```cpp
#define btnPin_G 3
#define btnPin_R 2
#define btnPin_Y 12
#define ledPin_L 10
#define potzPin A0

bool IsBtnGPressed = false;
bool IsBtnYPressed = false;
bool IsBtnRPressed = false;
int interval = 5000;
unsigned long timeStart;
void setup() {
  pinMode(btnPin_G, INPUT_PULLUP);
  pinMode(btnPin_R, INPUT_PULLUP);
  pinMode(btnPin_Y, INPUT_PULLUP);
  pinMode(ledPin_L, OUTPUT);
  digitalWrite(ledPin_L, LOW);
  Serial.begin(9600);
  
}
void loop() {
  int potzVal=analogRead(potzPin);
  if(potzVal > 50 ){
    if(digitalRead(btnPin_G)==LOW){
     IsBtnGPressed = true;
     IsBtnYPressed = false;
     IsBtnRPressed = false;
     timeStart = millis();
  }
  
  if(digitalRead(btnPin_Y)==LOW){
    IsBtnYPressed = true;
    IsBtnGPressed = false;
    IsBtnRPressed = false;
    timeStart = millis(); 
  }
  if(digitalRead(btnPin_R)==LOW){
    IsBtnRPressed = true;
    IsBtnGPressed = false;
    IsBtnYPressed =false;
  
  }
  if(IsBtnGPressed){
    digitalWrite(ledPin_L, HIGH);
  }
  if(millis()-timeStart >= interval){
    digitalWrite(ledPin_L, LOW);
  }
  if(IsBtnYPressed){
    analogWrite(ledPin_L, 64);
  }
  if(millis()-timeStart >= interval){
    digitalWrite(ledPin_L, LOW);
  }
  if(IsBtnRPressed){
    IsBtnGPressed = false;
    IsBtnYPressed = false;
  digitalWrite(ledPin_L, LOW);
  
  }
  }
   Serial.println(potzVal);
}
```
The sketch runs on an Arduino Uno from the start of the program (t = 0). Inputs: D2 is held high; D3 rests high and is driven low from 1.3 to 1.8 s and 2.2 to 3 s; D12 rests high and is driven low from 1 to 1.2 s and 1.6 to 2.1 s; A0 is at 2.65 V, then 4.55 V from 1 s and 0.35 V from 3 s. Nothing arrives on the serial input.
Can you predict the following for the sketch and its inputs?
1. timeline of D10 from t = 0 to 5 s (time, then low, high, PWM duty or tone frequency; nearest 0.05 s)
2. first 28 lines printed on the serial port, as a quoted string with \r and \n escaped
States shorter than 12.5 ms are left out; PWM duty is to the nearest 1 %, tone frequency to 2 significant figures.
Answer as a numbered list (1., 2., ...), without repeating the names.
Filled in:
1. 0 s low; 1 s PWM 25 %; 1.3 s high; 1.6 s PWM 25 %; 2.2 s high
2. "542\r\n542\r\n542\r\n542\r\n542\r\n542\r\n542\r\n542\r\n542\r\n542\r\n542\r\n542\r\n542\r\n542\r\n542\r\n542\r\n542\r\n542\r\n542\r\n542\r\n542\r\n542\r\n542\r\n542\r\n542\r\n542\r\n542\r\n542\r\n"
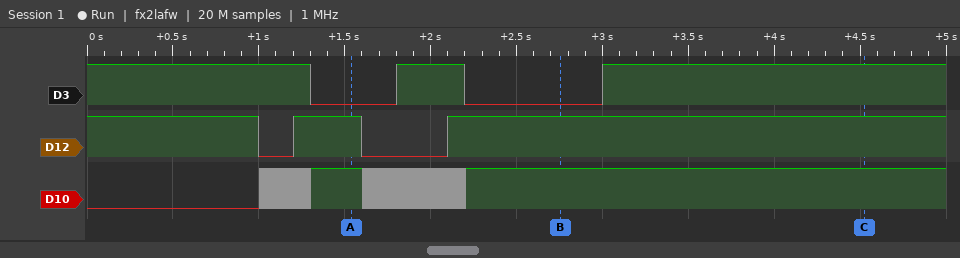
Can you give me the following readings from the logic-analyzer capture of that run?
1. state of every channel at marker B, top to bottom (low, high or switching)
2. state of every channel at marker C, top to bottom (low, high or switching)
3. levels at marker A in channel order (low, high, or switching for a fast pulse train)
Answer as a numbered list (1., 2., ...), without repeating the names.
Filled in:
1. D3 low, D12 high, D10 high
2. D3 high, D12 high, D10 high
3. D3 low, D12 high, D10 high
